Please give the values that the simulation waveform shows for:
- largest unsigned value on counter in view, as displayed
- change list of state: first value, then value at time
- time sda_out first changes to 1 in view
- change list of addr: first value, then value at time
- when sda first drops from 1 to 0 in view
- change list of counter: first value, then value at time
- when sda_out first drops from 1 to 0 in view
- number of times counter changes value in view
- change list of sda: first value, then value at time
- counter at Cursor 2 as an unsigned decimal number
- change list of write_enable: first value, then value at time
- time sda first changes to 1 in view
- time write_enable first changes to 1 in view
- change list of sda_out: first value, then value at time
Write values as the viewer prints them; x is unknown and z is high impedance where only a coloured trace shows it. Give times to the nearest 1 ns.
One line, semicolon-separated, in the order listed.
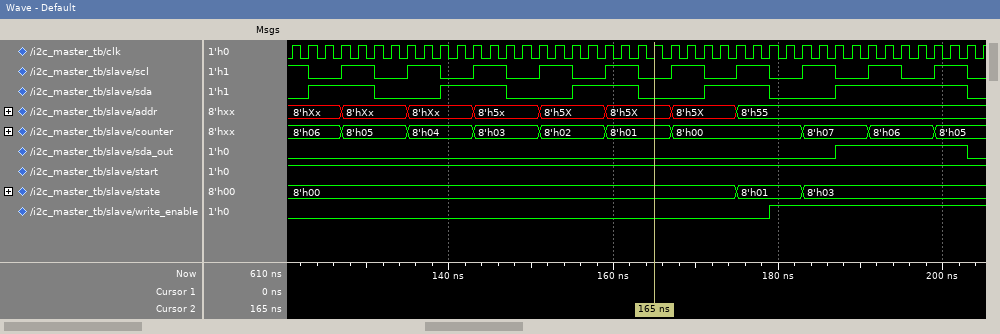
8'h07; 8'h00, 8'h01 at 175 ns, 8'h03 at 183 ns; 187 ns; 8'hXx, 8'hXx at 127 ns, 8'hXx at 135 ns, 8'h5x at 143 ns, 8'h5X at 151 ns, 8'h5X at 159 ns, 8'h5X at 167 ns, 8'h55 at 175 ns; 131 ns; 8'h06, 8'h05 at 127 ns, 8'h04 at 135 ns, 8'h03 at 143 ns, 8'h02 at 151 ns, 8'h01 at 159 ns, 8'h00 at 167 ns, 8'h07 at 183 ns, 8'h06 at 191 ns, 8'h05 at 199 ns; 203 ns; 9; 0, 1 at 123 ns, 0 at 131 ns, 1 at 139 ns, 0 at 147 ns, 1 at 155 ns, 0 at 163 ns, 1 at 171 ns, 0 at 179 ns, 1 at 187 ns, 0 at 203 ns; 1; 0, 1 at 179 ns; 123 ns; 179 ns; 0, 1 at 187 ns, 0 at 203 ns
